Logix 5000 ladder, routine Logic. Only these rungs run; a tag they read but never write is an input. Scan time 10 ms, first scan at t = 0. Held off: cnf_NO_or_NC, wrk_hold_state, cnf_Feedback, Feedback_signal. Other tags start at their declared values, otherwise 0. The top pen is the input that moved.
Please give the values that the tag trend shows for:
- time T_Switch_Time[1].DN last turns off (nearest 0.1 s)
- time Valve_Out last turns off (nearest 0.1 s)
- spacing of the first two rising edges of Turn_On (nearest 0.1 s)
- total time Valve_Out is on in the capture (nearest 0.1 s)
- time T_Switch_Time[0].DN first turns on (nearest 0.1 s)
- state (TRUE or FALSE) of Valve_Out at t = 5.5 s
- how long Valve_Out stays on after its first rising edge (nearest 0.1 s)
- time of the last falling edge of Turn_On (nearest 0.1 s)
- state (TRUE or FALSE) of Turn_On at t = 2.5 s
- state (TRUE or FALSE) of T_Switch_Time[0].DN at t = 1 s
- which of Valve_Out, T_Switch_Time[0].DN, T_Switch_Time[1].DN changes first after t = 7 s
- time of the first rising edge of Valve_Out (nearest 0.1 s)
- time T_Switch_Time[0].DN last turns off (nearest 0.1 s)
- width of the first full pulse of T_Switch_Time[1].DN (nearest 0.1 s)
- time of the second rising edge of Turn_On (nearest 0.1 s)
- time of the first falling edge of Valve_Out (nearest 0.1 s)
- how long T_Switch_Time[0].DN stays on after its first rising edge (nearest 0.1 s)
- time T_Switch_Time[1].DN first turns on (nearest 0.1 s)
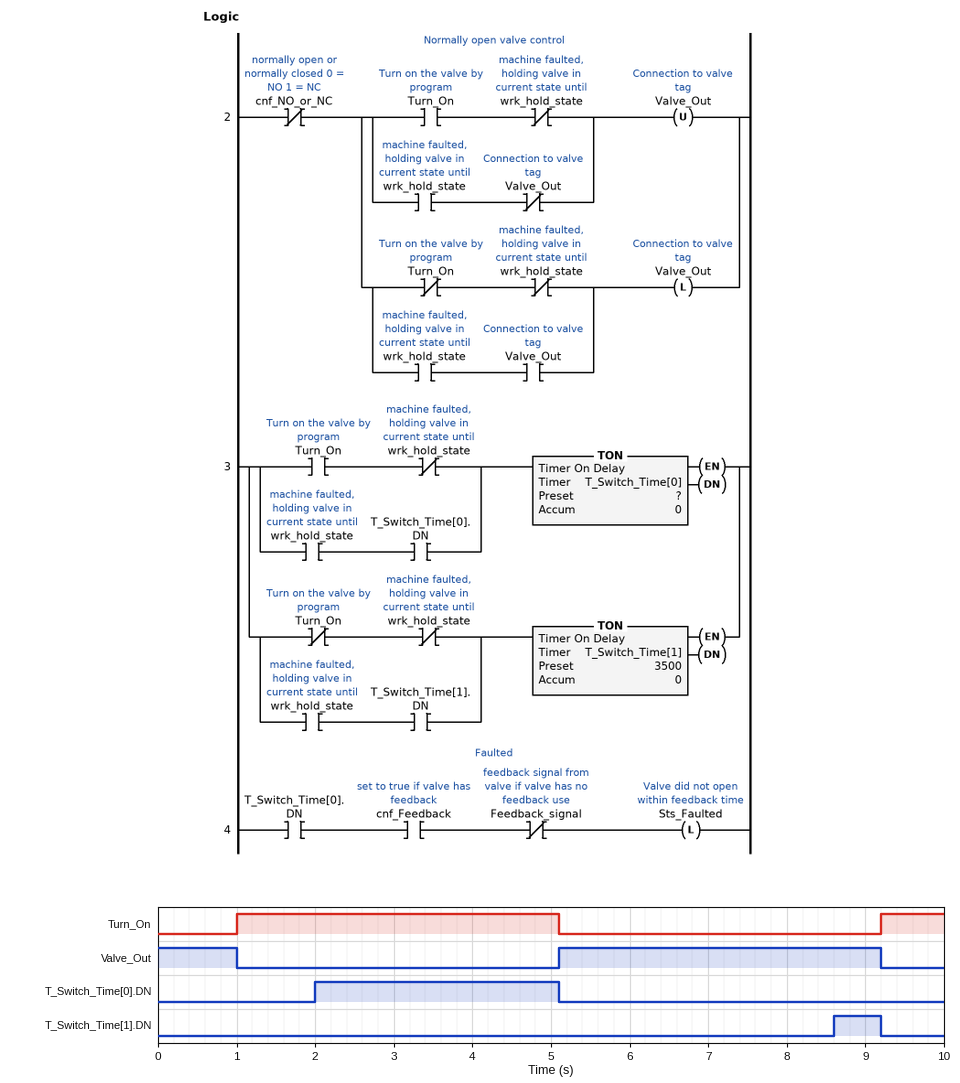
9.2 s
9.2 s
8.2 s
5.1 s
2.0 s
TRUE
4.1 s
5.1 s
TRUE
FALSE
T_Switch_Time[1].DN
5.1 s
5.1 s
0.6 s
9.2 s
1.0 s
3.1 s
8.6 s
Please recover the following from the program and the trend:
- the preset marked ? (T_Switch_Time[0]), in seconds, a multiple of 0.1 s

1.0 s
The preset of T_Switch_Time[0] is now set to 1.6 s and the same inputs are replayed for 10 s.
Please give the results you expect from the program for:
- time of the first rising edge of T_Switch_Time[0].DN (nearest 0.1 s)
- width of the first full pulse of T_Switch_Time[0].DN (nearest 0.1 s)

2.6 s
2.5 s
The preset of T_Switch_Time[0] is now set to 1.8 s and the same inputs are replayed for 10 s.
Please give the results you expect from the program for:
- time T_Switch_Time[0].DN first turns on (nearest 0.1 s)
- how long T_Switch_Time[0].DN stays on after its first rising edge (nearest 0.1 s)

2.8 s
2.3 s
